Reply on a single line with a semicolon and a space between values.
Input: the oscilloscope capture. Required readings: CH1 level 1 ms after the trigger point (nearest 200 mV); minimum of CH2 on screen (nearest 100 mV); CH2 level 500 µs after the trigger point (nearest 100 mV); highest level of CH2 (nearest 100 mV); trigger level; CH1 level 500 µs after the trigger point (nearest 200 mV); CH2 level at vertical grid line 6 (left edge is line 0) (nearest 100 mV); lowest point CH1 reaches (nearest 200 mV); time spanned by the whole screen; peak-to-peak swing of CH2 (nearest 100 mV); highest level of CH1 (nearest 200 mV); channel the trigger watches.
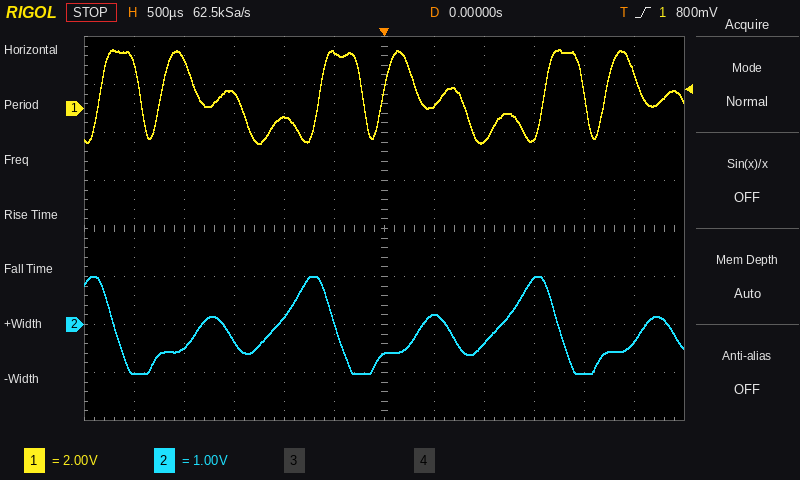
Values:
-1.4 V; -1.0 V; 200 mV; 1.0 V; 800 mV; 200 mV; -600 mV; -1.4 V; 6 ms; 2.0 V; 2.4 V; CH1
